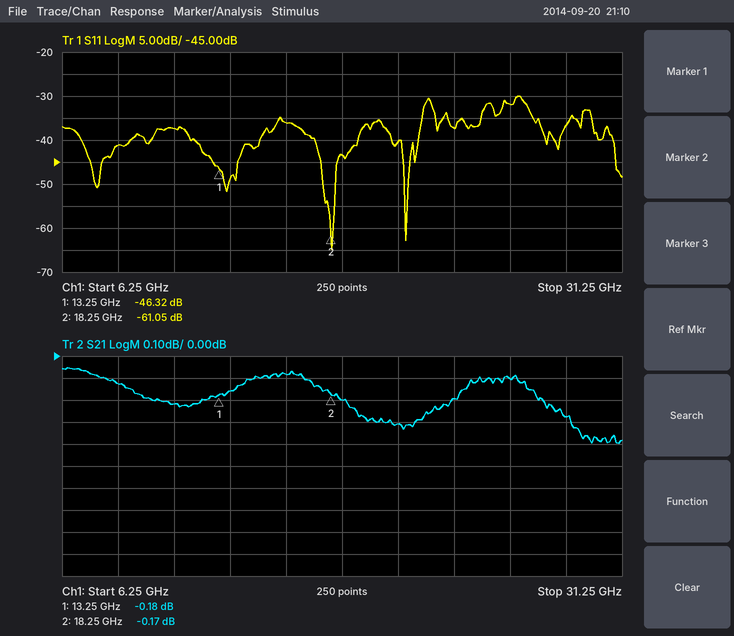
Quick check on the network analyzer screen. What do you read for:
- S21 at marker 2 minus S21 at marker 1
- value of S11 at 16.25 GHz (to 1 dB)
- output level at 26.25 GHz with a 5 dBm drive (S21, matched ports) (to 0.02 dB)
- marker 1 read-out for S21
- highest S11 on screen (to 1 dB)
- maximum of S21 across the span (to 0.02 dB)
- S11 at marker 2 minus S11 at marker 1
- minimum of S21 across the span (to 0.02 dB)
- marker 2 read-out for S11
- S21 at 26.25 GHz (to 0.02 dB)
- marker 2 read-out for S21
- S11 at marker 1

0.01 dB
-36 dB
4.90 dBm
-0.18 dB
-30 dB
-0.06 dB
-14.73 dB
-0.40 dB
-61.05 dB
-0.10 dB
-0.17 dB
-46.32 dB
